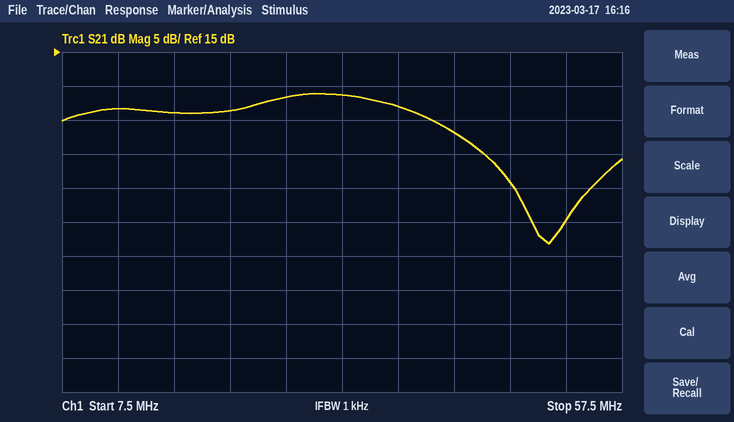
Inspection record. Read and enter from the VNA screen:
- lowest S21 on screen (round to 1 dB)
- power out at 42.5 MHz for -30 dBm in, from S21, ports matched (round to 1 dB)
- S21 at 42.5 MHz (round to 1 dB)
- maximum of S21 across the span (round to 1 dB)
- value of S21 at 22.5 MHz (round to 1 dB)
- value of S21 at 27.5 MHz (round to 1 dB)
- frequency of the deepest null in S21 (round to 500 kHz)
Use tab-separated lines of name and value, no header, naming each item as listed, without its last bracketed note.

lowest S21 on screen	-13 dB
power out at 42.5 MHz for -30 dBm in, from S21, ports matched	-27 dBm
S21 at 42.5 MHz	3 dB
maximum of S21 across the span	9 dB
value of S21 at 22.5 MHz	6 dB
value of S21 at 27.5 MHz	8 dB
frequency of the deepest null in S21	51.0 MHz
